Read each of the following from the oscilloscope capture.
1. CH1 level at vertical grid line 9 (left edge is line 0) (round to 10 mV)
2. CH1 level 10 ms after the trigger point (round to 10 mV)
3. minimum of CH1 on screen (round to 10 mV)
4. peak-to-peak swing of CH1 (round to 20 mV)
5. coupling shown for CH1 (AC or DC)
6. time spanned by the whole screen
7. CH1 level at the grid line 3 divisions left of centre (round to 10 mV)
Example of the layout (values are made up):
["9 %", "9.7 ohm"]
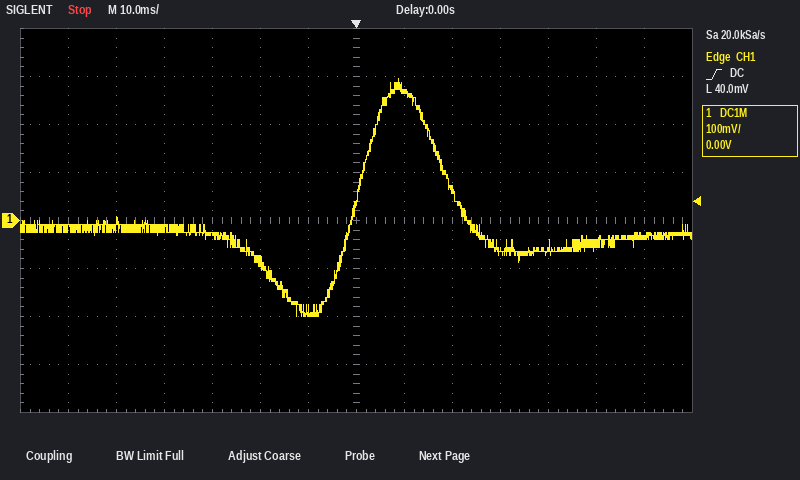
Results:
["60 mV", "270 mV", "-200 mV", "500 mV", "DC", "140 ms", "-30 mV"]
